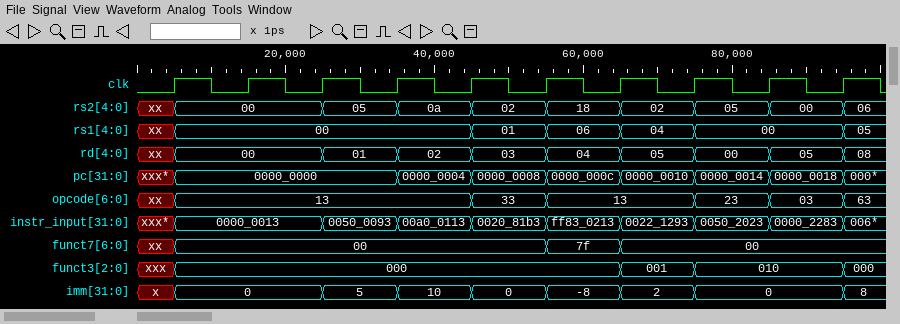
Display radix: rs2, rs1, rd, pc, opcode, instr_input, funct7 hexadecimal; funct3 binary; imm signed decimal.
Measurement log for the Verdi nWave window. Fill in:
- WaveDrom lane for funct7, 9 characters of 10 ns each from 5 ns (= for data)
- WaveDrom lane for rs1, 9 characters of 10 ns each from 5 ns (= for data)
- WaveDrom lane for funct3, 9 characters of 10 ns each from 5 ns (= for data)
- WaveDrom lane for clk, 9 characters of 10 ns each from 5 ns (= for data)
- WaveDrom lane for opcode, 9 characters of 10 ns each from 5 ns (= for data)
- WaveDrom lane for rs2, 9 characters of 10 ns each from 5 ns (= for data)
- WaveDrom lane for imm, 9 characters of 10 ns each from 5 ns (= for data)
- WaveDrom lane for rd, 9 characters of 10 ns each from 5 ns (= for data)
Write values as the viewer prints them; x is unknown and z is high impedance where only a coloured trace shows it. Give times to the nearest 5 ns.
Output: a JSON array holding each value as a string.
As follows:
["{name: 'funct7', wave: '=....==..', data: '00 7f 00'}", "{name: 'rs1', wave: '=...====.', data: '00 01 06 04 00'}", "{name: 'funct3', wave: '=.....==.', data: '000 001 010'}", "{name: 'clk', wave: 'p........'}", "{name: 'opcode', wave: '=...==.==', data: '13 33 13 23 03'}", "{name: 'rs2', wave: '=.=======', data: '00 05 0a 02 18 02 05 00'}", "{name: 'imm', wave: '=.======.', data: '0 5 10 0 -8 2 0'}", "{name: 'rd', wave: '=.=======', data: '00 01 02 03 04 05 00 05'}"]
